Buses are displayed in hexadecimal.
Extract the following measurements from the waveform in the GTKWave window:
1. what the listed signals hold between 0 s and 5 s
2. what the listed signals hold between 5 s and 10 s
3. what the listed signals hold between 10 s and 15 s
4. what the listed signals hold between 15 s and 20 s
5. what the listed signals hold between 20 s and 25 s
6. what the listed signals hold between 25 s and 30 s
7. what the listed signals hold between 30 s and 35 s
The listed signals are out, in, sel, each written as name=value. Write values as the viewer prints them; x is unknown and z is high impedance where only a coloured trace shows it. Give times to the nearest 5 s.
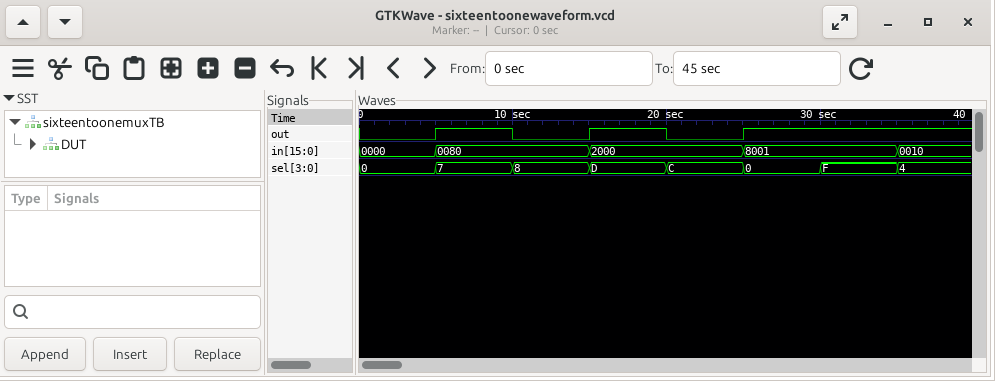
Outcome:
out=0, in=0000, sel=0
out=1, in=0080, sel=7
out=0, in=0080, sel=8
out=1, in=2000, sel=D
out=0, in=2000, sel=C
out=1, in=8001, sel=0
out=1, in=8001, sel=F
